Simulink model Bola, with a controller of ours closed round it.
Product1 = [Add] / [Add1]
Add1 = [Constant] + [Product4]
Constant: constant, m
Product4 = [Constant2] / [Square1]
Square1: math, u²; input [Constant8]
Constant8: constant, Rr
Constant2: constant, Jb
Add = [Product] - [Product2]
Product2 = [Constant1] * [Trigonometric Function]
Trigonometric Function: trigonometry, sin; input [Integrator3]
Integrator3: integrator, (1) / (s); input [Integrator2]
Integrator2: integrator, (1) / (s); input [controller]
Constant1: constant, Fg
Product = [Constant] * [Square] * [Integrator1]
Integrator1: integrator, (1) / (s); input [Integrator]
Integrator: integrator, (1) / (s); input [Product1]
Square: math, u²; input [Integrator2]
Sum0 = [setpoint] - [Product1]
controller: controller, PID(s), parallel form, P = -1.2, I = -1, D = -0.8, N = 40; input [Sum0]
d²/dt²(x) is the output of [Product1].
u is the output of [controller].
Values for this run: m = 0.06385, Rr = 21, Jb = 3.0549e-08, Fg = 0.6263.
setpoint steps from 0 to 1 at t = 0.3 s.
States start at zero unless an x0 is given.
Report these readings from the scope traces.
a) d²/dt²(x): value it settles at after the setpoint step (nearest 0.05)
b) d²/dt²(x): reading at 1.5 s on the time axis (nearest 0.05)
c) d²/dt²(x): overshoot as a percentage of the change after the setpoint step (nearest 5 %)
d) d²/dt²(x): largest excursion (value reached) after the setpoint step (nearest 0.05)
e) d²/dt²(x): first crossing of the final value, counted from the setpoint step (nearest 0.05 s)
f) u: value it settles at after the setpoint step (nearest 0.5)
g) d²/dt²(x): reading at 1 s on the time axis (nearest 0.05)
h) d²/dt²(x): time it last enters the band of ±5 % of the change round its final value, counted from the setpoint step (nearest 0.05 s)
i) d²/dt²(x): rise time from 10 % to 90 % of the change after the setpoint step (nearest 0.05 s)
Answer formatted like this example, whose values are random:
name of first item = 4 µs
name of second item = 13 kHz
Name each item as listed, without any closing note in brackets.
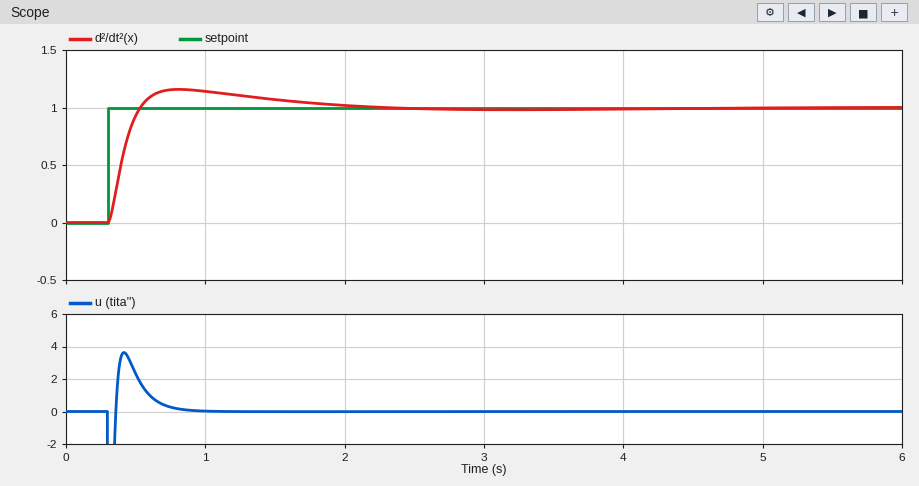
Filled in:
d²/dt²(x): value it settles at after the setpoint step = 1.00
d²/dt²(x): reading at 1.5 s on the time axis = 1.05
d²/dt²(x): overshoot as a percentage of the change after the setpoint step = 15 %
d²/dt²(x): largest excursion (value reached) after the setpoint step = 1.15
d²/dt²(x): first crossing of the final value, counted from the setpoint step = 0.25 s
u: value it settles at after the setpoint step = 0.0
d²/dt²(x): reading at 1 s on the time axis = 1.15
d²/dt²(x): time it last enters the band of ±5 % of the change round its final value, counted from the setpoint step = 1.35 s
d²/dt²(x): rise time from 10 % to 90 % of the change after the setpoint step = 0.15 s
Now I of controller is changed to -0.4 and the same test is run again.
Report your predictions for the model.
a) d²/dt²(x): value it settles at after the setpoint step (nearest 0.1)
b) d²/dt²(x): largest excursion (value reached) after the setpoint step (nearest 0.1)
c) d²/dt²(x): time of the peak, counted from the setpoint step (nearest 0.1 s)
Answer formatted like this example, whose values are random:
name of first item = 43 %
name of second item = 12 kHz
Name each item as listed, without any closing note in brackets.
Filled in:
d²/dt²(x): value it settles at after the setpoint step = 1.0
d²/dt²(x): largest excursion (value reached) after the setpoint step = 1.1
d²/dt²(x): time of the peak, counted from the setpoint step = 0.5 s
